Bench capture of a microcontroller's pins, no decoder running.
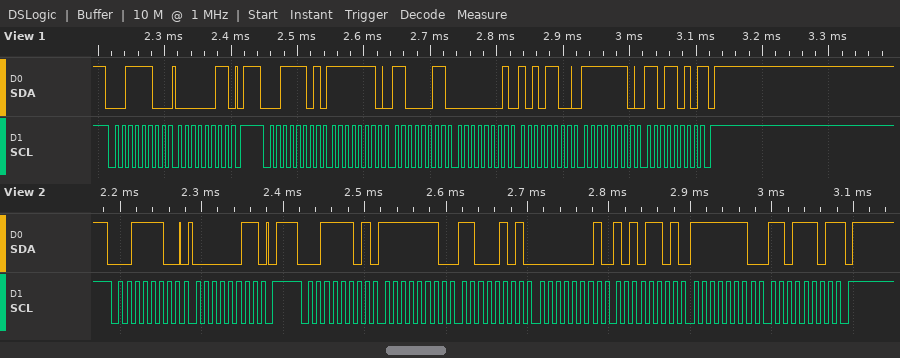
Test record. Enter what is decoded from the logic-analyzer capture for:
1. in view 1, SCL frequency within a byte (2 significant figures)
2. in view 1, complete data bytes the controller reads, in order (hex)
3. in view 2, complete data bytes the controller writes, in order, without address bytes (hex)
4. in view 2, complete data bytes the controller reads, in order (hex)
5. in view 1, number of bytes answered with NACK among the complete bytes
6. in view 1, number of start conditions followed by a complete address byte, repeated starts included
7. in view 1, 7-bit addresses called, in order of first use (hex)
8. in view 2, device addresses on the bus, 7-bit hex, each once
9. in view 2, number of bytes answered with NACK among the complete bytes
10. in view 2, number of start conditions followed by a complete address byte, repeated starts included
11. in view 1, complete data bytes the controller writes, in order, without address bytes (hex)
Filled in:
100 kHz
FE C3 01 AC FE DA
03
FE C5 01 AD FE DD
1
2
0x1E
0x1E
1
2
03
